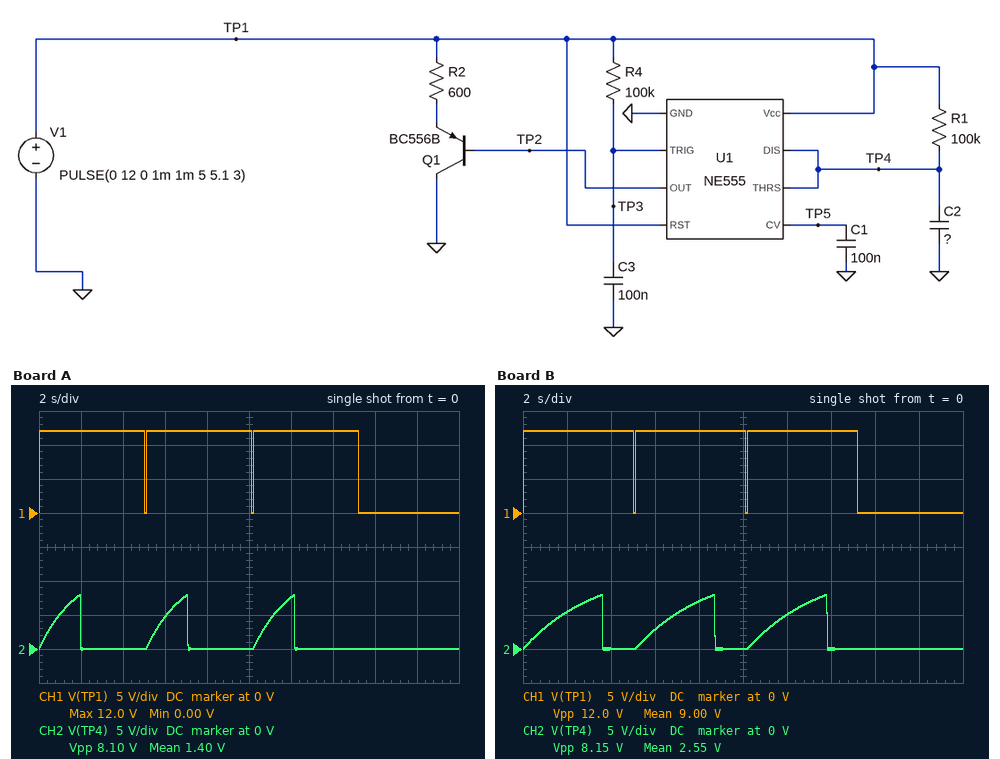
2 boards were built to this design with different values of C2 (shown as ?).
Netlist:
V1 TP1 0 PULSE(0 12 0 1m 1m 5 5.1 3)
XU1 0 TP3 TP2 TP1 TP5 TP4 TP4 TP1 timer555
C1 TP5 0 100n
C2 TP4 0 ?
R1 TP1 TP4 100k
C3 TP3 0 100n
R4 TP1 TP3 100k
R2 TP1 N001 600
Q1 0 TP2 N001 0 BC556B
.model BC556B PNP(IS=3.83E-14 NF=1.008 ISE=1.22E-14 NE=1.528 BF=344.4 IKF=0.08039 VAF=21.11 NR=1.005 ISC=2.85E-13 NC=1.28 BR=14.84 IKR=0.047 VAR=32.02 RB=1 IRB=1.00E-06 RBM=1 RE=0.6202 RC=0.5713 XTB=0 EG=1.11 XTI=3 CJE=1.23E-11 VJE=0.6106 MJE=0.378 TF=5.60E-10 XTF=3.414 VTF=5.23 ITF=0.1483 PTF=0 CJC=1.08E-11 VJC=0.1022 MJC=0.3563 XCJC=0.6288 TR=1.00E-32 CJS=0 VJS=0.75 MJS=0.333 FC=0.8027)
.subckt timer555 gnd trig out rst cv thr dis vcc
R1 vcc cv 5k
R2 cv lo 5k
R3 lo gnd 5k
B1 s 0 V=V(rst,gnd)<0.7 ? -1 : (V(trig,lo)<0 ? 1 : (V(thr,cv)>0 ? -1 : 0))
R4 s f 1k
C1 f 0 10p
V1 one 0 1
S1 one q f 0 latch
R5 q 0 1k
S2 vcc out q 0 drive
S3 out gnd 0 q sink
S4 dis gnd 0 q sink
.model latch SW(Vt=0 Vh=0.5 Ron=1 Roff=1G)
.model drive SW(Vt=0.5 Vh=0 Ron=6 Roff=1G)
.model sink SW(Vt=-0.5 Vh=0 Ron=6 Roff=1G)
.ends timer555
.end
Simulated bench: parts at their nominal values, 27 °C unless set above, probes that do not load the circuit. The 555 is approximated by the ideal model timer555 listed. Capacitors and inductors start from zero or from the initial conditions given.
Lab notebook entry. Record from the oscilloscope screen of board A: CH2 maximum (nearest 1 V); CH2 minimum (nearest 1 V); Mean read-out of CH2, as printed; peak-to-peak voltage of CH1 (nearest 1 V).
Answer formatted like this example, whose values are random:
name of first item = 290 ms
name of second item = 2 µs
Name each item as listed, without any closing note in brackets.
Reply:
CH2 maximum = 8 V
CH2 minimum = 0 V
Mean read-out of CH2, as printed = 1.40 V
peak-to-peak voltage of CH1 = 12 V
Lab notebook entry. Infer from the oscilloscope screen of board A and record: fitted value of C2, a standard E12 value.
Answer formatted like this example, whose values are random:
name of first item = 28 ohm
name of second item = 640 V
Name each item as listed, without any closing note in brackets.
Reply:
fitted value of C2, a standard E12 value = 18 µF
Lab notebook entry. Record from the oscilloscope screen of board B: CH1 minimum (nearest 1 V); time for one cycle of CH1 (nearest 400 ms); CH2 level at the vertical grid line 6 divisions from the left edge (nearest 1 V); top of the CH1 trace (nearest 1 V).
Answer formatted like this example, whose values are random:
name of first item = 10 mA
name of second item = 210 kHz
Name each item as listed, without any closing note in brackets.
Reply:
CH1 minimum = 0 V
time for one cycle of CH1 = 5.2 s
CH2 level at the vertical grid line 6 divisions from the left edge = 5 V
top of the CH1 trace = 12 V
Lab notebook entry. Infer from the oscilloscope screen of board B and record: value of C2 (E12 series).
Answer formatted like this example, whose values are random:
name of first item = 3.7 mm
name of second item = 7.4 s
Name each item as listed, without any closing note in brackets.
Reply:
value of C2 = 33 µF
